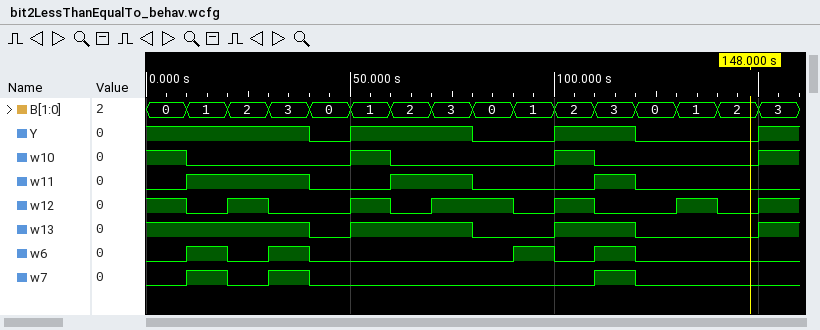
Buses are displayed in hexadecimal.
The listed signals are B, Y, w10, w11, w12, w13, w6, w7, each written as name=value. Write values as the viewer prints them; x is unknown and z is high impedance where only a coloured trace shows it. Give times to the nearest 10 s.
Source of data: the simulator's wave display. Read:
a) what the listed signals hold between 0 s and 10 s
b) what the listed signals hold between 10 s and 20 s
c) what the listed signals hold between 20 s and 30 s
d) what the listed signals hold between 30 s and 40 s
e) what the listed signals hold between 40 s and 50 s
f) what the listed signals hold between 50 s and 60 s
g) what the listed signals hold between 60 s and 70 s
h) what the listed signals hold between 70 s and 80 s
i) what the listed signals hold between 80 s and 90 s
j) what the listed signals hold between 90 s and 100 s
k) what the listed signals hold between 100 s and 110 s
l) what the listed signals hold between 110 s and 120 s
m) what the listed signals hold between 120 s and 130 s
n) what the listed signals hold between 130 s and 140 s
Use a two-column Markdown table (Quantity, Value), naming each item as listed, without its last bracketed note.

| Quantity | Value |
|---|---|
| what the listed signals hold between 0 s and 10 s | B=0, Y=1, w10=1, w11=0, w12=1, w13=1, w6=0, w7=0 |
| what the listed signals hold between 10 s and 20 s | B=1, Y=1, w10=0, w11=1, w12=0, w13=1, w6=1, w7=1 |
| what the listed signals hold between 20 s and 30 s | B=2, Y=1, w10=0, w11=1, w12=1, w13=1, w6=0, w7=0 |
| what the listed signals hold between 30 s and 40 s | B=3, Y=1, w10=0, w11=1, w12=0, w13=1, w6=1, w7=1 |
| what the listed signals hold between 40 s and 50 s | B=0, Y=0, w10=0, w11=0, w12=0, w13=0, w6=0, w7=0 |
| what the listed signals hold between 50 s and 60 s | B=1, Y=1, w10=1, w11=0, w12=1, w13=1, w6=0, w7=0 |
| what the listed signals hold between 60 s and 70 s | B=2, Y=1, w10=0, w11=1, w12=0, w13=1, w6=0, w7=0 |
| what the listed signals hold between 70 s and 80 s | B=3, Y=1, w10=0, w11=1, w12=1, w13=1, w6=0, w7=0 |
| what the listed signals hold between 80 s and 90 s | B=0, Y=0, w10=0, w11=0, w12=1, w13=0, w6=0, w7=0 |
| what the listed signals hold between 90 s and 100 s | B=1, Y=0, w10=0, w11=0, w12=0, w13=0, w6=1, w7=0 |
| what the listed signals hold between 100 s and 110 s | B=2, Y=1, w10=1, w11=0, w12=1, w13=1, w6=0, w7=0 |
| what the listed signals hold between 110 s and 120 s | B=3, Y=1, w10=0, w11=1, w12=0, w13=1, w6=1, w7=1 |
| what the listed signals hold between 120 s and 130 s | B=0, Y=0, w10=0, w11=0, w12=0, w13=0, w6=0, w7=0 |
| what the listed signals hold between 130 s and 140 s | B=1, Y=0, w10=0, w11=0, w12=1, w13=0, w6=0, w7=0 |
